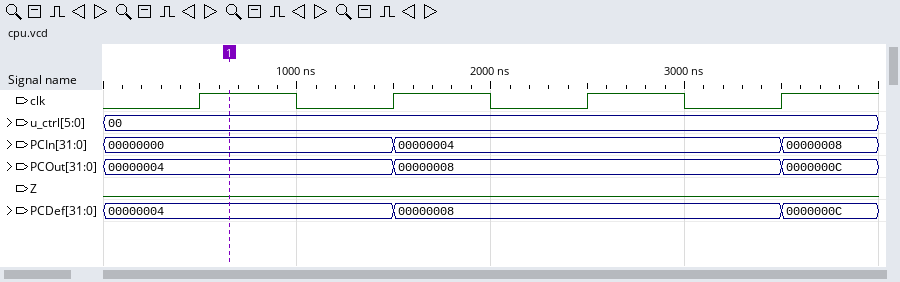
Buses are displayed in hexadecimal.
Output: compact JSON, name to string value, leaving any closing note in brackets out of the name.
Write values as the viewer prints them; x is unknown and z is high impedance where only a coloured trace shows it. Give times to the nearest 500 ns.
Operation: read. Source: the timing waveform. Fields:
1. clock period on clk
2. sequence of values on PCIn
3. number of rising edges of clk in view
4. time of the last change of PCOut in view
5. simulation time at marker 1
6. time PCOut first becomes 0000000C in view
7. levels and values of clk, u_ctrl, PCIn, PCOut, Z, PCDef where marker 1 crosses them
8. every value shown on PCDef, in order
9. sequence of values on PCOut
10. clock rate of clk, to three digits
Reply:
{"clock period on clk": "1000 ns", "sequence of values on PCIn": "00000000, 00000004, 00000008", "number of rising edges of clk in view": "4", "time of the last change of PCOut in view": "3500 ns", "simulation time at marker 1": "500 ns", "time PCOut first becomes 0000000C in view": "3500 ns", "levels and values of clk, u_ctrl, PCIn, PCOut, Z, PCDef where marker 1 crosses them": "clk=1, u_ctrl=00, PCIn=00000000, PCOut=00000004, Z=0, PCDef=00000004", "every value shown on PCDef, in order": "00000004, 00000008, 0000000C", "sequence of values on PCOut": "00000004, 00000008, 0000000C", "clock rate of clk, to three digits": "1.00 MHz"}
